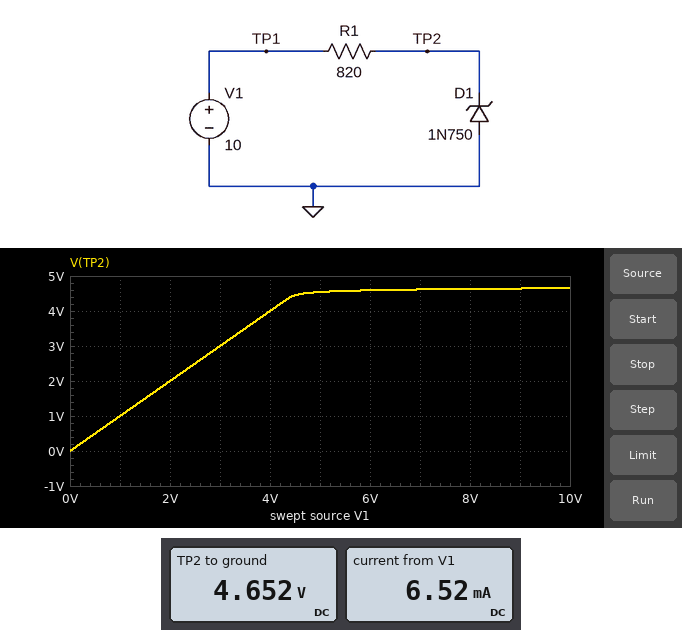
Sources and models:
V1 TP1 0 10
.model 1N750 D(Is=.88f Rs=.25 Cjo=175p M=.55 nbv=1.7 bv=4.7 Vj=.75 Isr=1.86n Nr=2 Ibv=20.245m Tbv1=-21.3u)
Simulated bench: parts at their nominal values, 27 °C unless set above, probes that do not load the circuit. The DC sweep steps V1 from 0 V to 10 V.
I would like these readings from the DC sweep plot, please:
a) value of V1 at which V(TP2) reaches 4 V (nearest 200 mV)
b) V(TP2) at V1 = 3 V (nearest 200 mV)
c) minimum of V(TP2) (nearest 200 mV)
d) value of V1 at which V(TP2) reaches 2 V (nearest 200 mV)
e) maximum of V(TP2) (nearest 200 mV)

4.0 V
3.0 V
0 V
2.0 V
4.6 V
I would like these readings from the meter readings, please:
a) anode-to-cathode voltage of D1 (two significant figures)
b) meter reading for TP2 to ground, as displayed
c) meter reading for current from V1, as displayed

-4.7 V
4.652 V
6.52 mA
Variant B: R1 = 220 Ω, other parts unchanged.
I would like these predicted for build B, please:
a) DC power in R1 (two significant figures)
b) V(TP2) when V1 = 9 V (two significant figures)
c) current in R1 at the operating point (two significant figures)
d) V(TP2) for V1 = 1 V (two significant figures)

130 mW
4.7 V
24 mA
1.0 V
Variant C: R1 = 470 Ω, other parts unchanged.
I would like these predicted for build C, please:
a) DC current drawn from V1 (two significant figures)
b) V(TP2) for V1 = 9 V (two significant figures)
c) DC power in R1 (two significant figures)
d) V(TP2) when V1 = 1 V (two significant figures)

11 mA
4.7 V
60 mW
1.0 V
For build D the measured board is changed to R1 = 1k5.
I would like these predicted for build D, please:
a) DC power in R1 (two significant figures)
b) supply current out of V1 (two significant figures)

19 mW
3.6 mA
